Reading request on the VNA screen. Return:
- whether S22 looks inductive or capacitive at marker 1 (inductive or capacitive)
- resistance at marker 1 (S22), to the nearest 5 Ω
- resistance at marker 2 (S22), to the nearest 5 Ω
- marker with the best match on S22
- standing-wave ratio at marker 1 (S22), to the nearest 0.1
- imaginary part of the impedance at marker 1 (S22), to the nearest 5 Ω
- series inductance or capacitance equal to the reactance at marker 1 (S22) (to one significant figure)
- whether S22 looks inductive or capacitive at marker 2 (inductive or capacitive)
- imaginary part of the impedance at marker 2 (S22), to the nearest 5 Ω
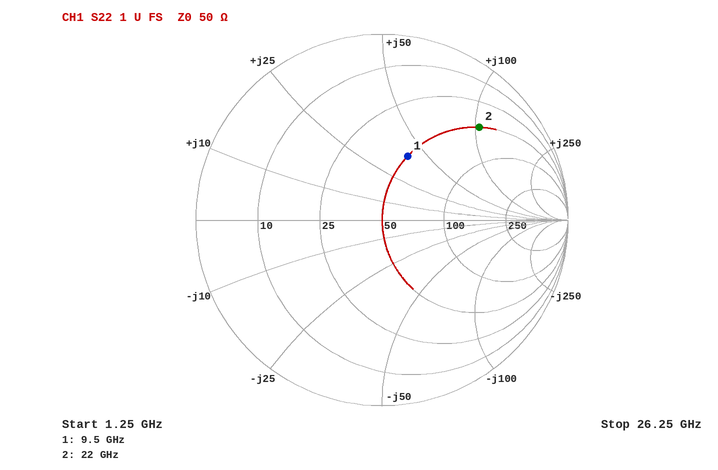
inductive
50 Ω
50 Ω
marker 1
2.2
+40 Ω
700 pH
inductive
+105 Ω
